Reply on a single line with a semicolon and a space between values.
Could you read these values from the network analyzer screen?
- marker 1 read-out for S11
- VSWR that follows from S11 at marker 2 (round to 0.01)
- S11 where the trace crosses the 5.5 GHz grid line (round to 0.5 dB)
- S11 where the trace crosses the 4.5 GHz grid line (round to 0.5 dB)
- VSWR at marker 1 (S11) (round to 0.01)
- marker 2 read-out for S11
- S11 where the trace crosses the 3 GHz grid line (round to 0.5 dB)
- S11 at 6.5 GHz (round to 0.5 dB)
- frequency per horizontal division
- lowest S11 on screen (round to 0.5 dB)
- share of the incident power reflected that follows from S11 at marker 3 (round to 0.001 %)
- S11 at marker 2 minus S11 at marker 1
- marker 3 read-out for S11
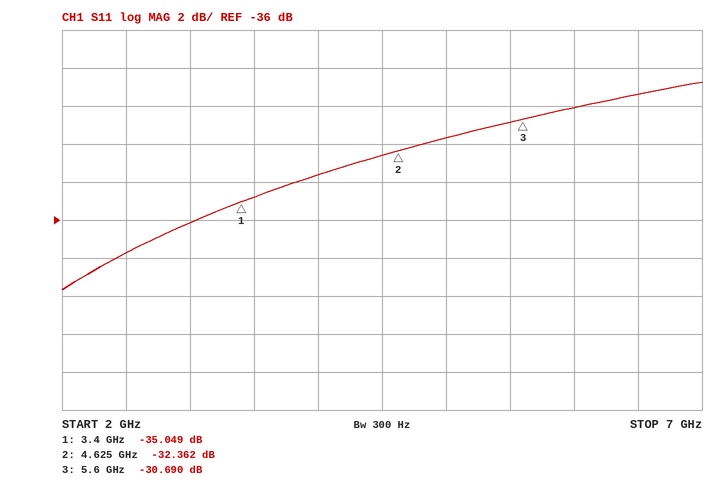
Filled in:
-35.049 dB; 1.05; -31.0 dB; -32.5 dB; 1.04; -32.362 dB; -36.0 dB; -29.5 dB; 500 MHz; -39.5 dB; 0.085 %; 2.687 dB; -30.690 dB
